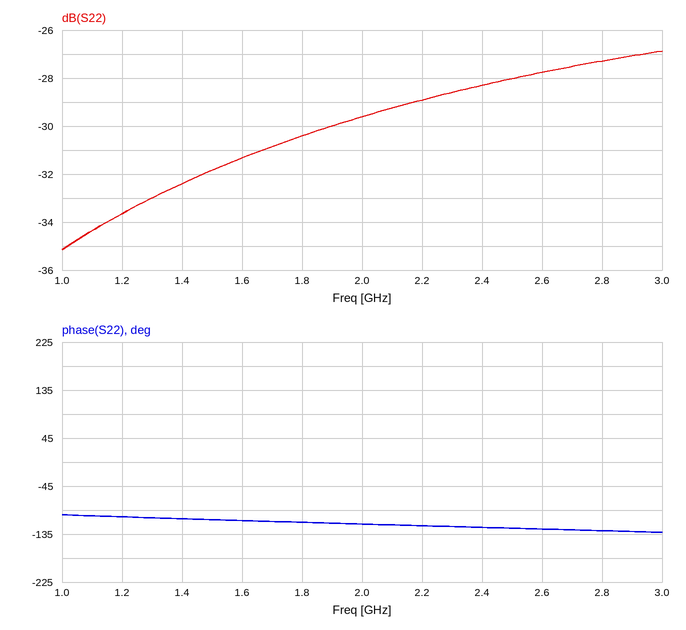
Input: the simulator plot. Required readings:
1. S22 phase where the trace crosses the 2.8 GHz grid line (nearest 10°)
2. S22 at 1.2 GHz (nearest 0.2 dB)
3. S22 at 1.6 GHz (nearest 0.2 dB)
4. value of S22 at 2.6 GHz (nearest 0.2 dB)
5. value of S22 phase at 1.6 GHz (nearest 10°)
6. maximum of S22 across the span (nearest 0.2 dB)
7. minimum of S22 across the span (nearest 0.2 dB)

-130°
-33.6 dB
-31.4 dB
-27.8 dB
-110°
-26.8 dB
-35.2 dB
